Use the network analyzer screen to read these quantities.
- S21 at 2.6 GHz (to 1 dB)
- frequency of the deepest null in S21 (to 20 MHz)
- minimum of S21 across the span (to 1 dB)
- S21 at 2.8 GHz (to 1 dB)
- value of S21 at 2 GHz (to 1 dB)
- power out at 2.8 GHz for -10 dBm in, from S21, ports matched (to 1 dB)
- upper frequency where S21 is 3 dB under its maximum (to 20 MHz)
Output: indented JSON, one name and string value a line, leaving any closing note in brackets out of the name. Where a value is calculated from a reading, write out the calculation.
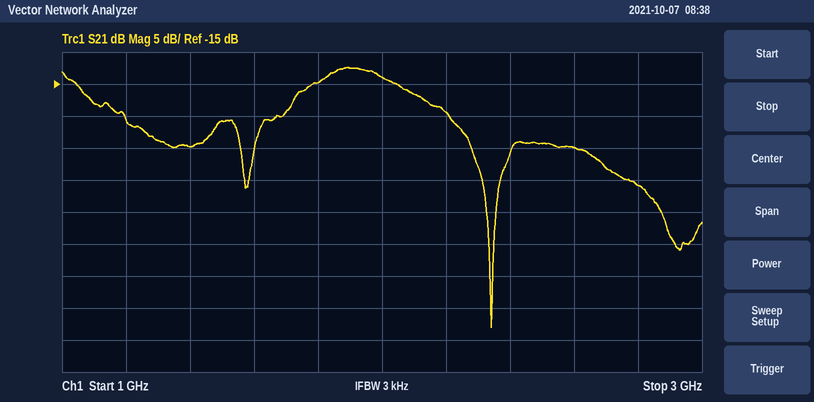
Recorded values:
{
  "S21 at 2.6 GHz": "-25 dB",
  "frequency of the deepest null in S21": "2.34 GHz",
  "minimum of S21 across the span": "-53 dB",
  "S21 at 2.8 GHz": "-31 dB",
  "value of S21 at 2 GHz": "-14 dB",
  "power out at 2.8 GHz for -10 dBm in, from S21, ports matched": "-10 dBm + (-31 dB) = -41 dBm",
  "upper frequency where S21 is 3 dB under its maximum": "2.06 GHz"
}
